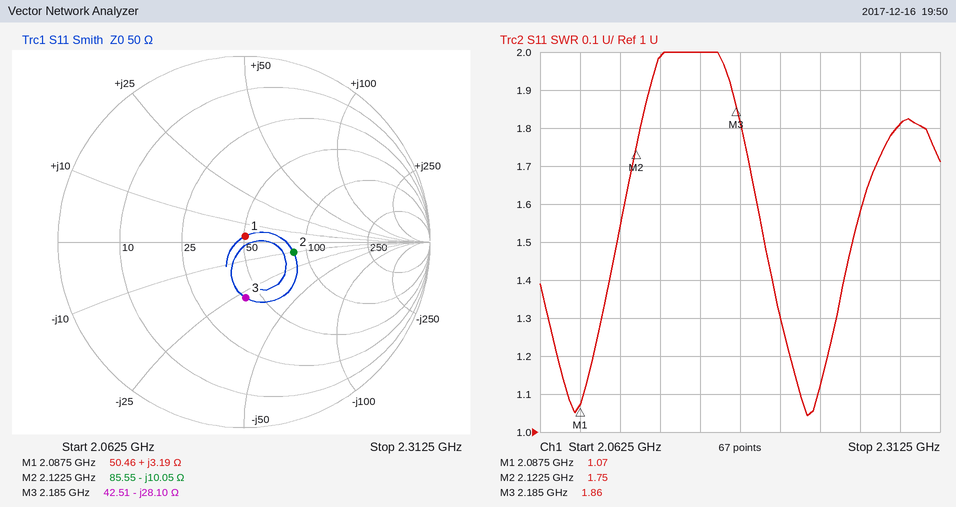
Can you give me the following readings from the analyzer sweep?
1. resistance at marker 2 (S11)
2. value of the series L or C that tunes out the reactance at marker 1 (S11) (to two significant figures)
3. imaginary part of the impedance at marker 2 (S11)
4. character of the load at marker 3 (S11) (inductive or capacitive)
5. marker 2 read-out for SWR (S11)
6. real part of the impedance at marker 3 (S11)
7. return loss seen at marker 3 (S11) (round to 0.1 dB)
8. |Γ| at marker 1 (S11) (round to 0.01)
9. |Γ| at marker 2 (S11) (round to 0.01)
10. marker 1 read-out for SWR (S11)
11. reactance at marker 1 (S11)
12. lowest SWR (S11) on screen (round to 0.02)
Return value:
85.55 Ω
24 pF
-10.05 Ω
capacitive
1.75
42.51 Ω
10.4 dB
0.03
0.27
1.07
+3.19 Ω
1.04
